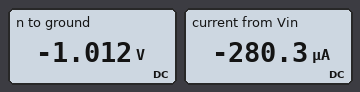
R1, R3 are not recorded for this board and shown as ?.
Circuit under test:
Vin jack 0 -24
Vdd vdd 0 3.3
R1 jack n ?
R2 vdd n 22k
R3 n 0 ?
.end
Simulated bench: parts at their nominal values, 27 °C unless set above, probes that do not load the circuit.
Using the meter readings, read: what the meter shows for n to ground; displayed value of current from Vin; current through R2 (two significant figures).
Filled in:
-1.012 V
-280.3 µA
200 µA
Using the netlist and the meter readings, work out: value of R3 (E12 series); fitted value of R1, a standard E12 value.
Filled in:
12 kΩ
82 kΩ
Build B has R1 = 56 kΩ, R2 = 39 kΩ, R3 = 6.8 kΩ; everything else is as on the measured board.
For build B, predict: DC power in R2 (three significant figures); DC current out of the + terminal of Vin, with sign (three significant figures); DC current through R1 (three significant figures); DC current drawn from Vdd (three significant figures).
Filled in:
668 µW
-396 µA
396 µA
131 µA
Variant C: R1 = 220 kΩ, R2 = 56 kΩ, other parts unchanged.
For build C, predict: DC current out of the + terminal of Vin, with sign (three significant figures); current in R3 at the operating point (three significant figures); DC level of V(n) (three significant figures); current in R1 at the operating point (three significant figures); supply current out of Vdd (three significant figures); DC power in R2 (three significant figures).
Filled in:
-107 µA
39.5 µA
-474 mV
107 µA
67.4 µA
254 µW
